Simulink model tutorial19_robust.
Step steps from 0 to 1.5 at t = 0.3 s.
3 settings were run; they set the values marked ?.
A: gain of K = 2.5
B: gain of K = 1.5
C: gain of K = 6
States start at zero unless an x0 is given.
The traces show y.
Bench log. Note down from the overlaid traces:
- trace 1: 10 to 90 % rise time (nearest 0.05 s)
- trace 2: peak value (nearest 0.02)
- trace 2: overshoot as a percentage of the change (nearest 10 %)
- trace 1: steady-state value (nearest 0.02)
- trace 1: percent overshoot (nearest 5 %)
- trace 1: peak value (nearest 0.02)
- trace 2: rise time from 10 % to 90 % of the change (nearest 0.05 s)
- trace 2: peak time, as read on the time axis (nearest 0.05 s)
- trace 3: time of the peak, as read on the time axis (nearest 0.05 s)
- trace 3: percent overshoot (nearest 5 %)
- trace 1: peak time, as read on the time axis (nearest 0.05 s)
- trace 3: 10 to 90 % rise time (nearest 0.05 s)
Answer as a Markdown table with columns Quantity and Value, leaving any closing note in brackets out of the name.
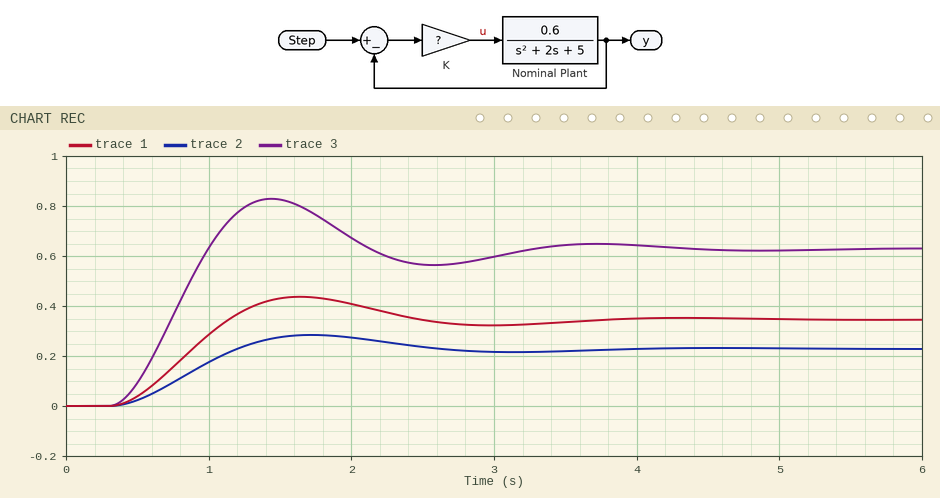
| Quantity | Value |
|---|---|
| trace 1: 10 to 90 % rise time | 0.55 s |
| trace 2: peak value | 0.28 |
| trace 2: overshoot as a percentage of the change | 20 % |
| trace 1: steady-state value | 0.34 |
| trace 1: percent overshoot | 25 % |
| trace 1: peak value | 0.44 |
| trace 2: rise time from 10 % to 90 % of the change | 0.60 s |
| trace 2: peak time, as read on the time axis | 1.70 s |
| trace 3: time of the peak, as read on the time axis | 1.45 s |
| trace 3: percent overshoot | 30 % |
| trace 1: peak time, as read on the time axis | 1.65 s |
| trace 3: 10 to 90 % rise time | 0.45 s |
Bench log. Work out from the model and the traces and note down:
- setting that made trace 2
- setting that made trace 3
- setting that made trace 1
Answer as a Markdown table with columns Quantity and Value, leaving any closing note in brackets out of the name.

| Quantity | Value |
|---|---|
| setting that made trace 2 | B |
| setting that made trace 3 | C |
| setting that made trace 1 | A |
